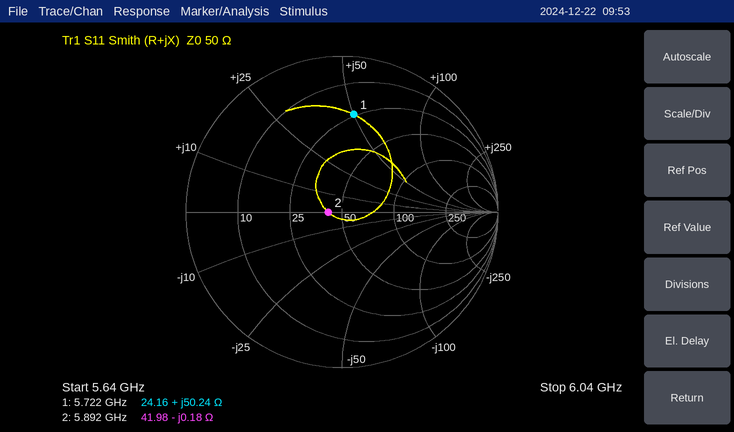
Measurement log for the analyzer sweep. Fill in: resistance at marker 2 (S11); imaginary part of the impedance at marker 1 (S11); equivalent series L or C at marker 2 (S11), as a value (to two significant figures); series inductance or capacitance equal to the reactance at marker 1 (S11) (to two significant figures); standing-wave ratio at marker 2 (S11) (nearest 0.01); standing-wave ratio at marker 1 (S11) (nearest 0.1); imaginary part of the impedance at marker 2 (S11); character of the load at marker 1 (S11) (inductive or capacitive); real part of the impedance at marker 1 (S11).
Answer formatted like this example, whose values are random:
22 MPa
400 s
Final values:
41.98 Ω
+50.24 Ω
150 pF
1.4 nH
1.19
4.4
-0.18 Ω
inductive
24.16 Ω
